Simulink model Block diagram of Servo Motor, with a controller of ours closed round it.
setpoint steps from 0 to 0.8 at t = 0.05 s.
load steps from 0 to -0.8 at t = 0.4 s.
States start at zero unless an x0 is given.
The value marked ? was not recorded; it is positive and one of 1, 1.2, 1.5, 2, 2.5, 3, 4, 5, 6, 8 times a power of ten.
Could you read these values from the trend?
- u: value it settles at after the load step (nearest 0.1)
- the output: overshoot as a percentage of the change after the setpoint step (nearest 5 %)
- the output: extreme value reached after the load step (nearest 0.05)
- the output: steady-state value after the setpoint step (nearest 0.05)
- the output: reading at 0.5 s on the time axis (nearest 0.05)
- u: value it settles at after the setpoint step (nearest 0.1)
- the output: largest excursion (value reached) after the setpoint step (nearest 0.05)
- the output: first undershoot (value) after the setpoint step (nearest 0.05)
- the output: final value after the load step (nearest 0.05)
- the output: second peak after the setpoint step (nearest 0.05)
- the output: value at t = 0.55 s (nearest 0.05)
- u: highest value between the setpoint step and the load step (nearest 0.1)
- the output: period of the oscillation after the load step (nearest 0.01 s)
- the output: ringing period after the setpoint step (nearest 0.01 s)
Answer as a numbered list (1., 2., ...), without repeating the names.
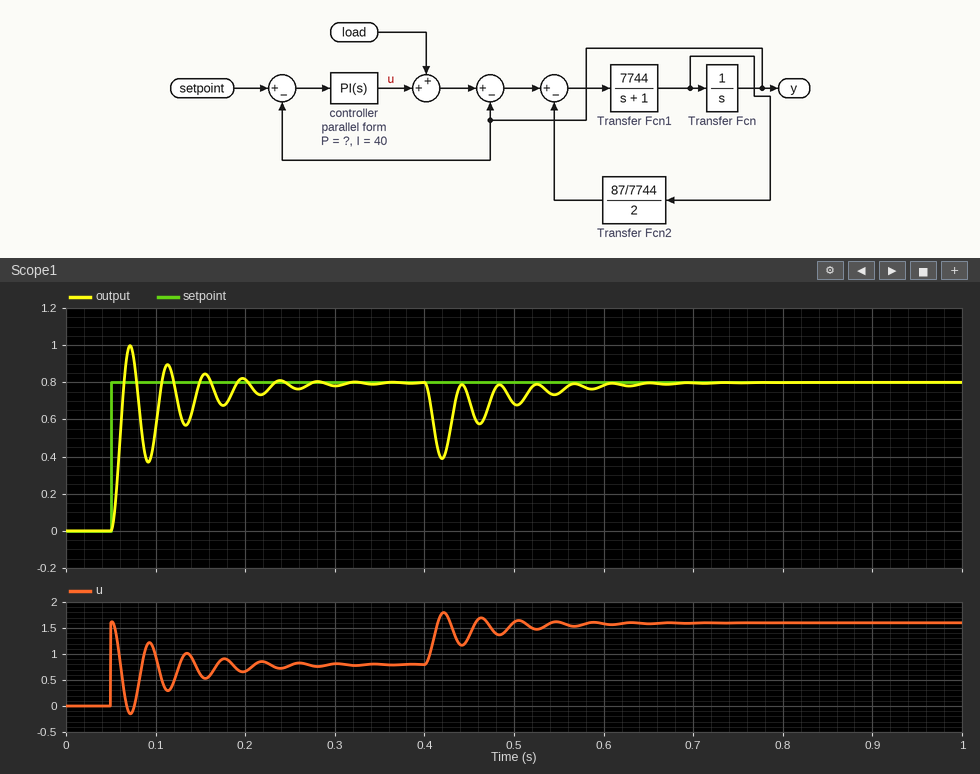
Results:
1. 1.6
2. 25 %
3. 0.40
4. 0.80
5. 0.70
6. 0.8
7. 1.00
8. 0.35
9. 0.80
10. 0.90
11. 0.75
12. 1.6
13. 0.04 s
14. 0.04 s
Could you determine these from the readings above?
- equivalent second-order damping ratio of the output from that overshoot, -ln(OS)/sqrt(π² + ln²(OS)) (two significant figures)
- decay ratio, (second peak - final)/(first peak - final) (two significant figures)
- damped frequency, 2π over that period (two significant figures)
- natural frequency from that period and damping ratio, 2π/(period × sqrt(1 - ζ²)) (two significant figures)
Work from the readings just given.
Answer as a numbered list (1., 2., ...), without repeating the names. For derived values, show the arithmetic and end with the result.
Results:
1. ln(0.25) = -1.386; 1.386 / sqrt(9.870 + 1.922) = 0.40
2. (0.9 - 0.8) / (1 - 0.8) = 0.50
3. 2π / 0.04 = 160 rad/s
4. 2π / (0.04 × sqrt(1 - 0.4²)) = 170 rad/s
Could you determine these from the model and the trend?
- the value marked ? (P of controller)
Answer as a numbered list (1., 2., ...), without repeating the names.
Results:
1. 2
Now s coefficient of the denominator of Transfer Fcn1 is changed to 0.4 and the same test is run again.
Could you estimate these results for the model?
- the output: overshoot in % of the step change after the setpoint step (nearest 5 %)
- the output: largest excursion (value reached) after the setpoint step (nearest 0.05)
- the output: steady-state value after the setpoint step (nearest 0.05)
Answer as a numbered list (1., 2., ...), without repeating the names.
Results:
1. 10 %
2. 0.85
3. 0.80
